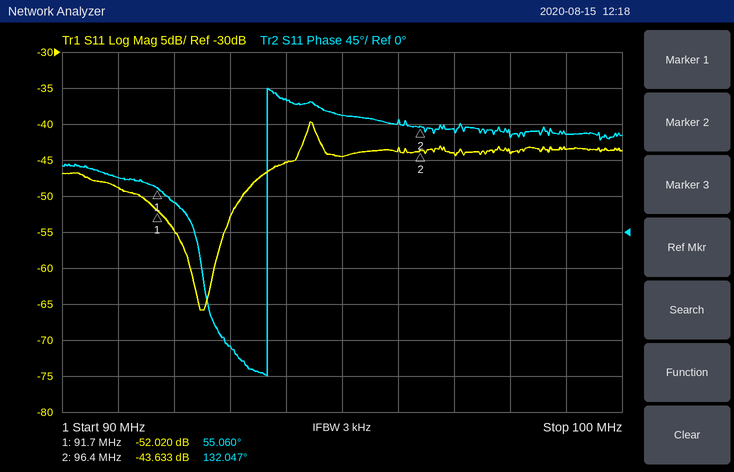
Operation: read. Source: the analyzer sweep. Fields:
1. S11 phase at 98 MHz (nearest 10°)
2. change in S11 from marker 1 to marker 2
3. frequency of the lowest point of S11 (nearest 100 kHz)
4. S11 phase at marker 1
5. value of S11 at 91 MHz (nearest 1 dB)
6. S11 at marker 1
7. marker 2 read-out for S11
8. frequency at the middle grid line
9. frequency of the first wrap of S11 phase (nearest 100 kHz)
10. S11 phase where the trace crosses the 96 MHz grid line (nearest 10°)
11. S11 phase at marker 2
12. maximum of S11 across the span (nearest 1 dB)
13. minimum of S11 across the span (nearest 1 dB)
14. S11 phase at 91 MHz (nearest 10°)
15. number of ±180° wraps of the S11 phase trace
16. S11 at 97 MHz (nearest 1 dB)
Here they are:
120°
8.387 dB
92.5 MHz
55.060°
-49 dB
-52.020 dB
-43.633 dB
95 MHz
93.7 MHz
140°
132.047°
-40 dB
-66 dB
70°
1
-44 dB
